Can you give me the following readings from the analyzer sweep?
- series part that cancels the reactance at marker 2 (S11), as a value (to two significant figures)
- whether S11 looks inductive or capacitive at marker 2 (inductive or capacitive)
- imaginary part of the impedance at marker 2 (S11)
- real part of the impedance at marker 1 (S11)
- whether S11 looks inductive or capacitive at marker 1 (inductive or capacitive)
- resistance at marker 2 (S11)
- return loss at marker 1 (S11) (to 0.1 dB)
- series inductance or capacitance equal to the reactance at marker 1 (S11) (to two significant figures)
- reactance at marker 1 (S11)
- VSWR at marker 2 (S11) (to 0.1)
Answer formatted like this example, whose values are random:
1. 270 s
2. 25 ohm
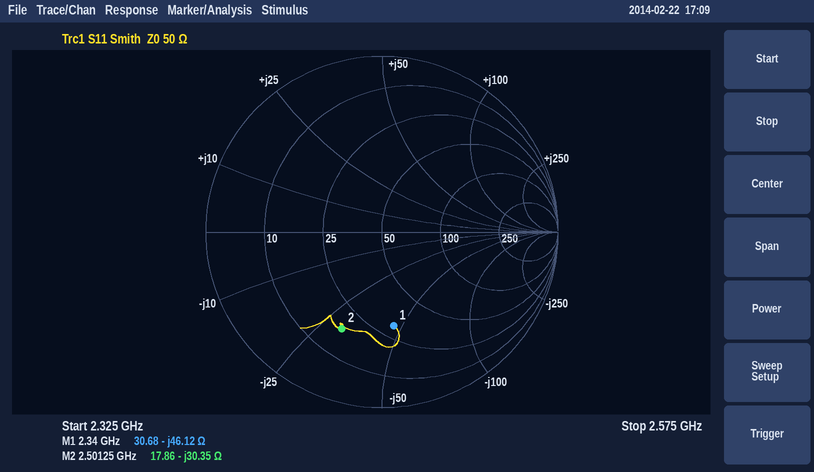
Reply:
1. 1.9 nH
2. capacitive
3. -30.35 Ω
4. 30.68 Ω
5. capacitive
6. 17.86 Ω
7. 5.4 dB
8. 1.5 pF
9. -46.12 Ω
10. 3.9
